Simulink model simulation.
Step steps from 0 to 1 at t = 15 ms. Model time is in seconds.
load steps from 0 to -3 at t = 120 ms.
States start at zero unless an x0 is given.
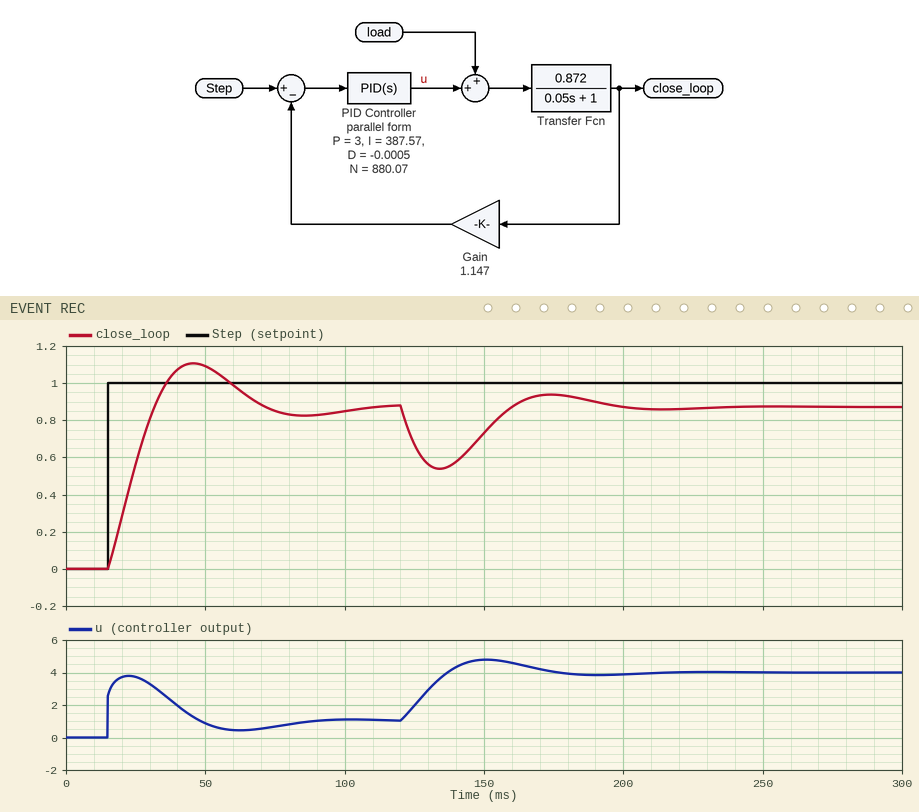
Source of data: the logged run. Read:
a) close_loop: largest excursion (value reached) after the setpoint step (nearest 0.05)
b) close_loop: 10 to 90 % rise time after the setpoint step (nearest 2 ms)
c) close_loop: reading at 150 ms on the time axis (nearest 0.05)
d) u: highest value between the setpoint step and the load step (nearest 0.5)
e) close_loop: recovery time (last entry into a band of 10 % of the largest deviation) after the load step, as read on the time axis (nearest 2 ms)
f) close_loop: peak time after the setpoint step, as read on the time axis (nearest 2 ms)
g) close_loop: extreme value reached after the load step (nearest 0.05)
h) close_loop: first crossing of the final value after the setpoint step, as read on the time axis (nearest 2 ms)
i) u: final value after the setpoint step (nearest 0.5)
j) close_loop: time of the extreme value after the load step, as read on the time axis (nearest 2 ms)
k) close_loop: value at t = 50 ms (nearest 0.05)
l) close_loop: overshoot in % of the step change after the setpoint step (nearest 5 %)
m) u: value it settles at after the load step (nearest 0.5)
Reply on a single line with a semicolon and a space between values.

1.10; 12 ms; 0.75; 4.0; 188 ms; 46 ms; 0.55; 32 ms; 1.0; 134 ms; 1.10; 25 %; 4.0
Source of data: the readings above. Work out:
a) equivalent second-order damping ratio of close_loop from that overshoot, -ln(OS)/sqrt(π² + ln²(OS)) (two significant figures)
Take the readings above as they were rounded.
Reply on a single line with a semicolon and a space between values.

0.40
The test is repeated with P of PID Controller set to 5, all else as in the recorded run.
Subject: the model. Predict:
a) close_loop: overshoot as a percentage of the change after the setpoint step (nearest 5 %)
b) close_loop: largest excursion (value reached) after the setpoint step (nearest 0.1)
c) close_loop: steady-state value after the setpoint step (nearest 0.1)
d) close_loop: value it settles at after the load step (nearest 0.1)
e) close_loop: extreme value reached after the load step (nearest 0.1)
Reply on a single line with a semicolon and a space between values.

15 %; 1.0; 0.9; 0.9; 0.6
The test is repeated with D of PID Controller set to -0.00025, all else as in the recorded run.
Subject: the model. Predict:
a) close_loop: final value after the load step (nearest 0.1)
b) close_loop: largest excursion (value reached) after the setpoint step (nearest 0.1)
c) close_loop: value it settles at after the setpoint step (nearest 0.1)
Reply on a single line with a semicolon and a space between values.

0.9; 1.1; 0.9
